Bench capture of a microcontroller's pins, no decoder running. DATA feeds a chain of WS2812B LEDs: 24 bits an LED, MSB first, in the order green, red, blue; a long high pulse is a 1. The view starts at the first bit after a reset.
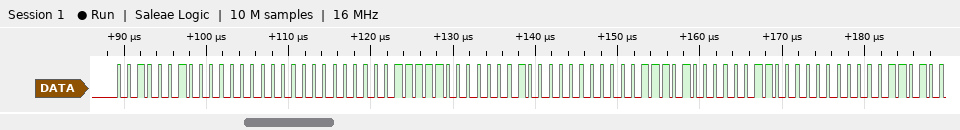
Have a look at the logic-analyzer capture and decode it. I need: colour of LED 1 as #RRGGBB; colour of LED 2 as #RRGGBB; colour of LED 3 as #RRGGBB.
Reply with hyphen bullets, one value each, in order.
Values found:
- #002200
- #011F00
- #031D00
